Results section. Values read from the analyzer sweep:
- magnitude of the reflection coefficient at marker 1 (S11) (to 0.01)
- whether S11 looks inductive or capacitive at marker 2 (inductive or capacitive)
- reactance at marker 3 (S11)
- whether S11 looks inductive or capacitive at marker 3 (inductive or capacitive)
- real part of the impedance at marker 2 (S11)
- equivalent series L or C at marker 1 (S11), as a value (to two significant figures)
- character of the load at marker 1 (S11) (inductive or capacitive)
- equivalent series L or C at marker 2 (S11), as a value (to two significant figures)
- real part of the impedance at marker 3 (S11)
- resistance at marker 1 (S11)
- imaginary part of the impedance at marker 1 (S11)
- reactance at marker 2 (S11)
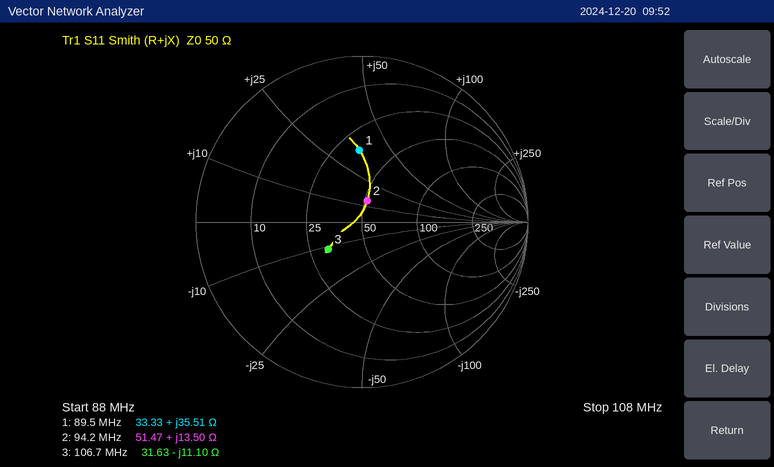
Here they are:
0.43
inductive
-11.10 Ω
capacitive
51.47 Ω
63 nH
inductive
23 nH
31.63 Ω
33.33 Ω
+35.51 Ω
+13.50 Ω
